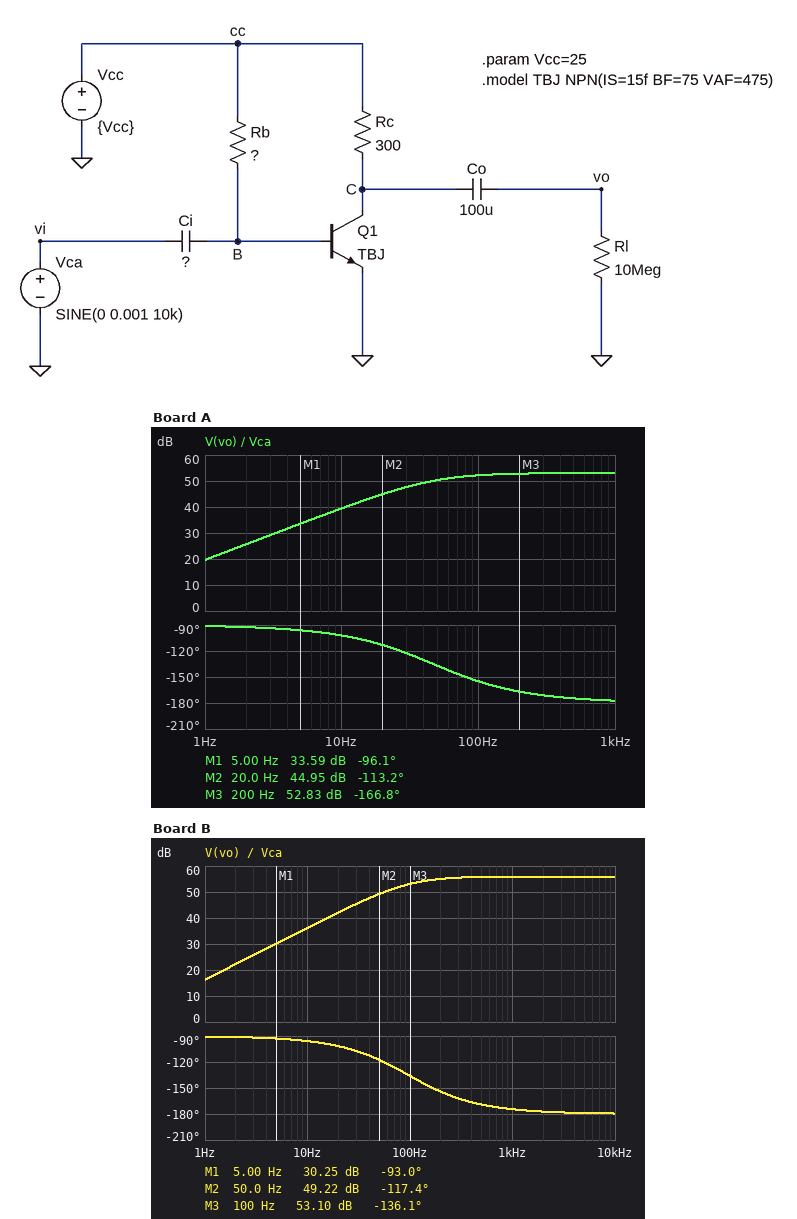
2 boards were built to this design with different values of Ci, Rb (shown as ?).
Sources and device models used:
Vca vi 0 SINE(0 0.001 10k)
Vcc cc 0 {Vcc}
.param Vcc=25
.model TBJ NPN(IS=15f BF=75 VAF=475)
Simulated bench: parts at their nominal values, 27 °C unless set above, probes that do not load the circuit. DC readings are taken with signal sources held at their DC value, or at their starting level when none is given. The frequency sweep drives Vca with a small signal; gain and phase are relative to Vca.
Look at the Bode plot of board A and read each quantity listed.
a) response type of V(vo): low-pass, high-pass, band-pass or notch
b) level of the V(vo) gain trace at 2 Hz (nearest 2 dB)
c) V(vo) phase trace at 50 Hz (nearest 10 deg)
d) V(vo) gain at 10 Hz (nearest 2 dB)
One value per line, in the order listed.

high-pass
26 dB
-140 deg
40 dB
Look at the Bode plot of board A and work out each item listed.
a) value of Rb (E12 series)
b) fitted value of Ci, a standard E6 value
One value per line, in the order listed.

47 kΩ
68 µF
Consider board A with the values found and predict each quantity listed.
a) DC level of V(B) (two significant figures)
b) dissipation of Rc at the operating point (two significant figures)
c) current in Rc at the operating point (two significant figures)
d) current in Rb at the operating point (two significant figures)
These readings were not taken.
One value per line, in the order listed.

740 mV
470 mW
40 mA
520 µA
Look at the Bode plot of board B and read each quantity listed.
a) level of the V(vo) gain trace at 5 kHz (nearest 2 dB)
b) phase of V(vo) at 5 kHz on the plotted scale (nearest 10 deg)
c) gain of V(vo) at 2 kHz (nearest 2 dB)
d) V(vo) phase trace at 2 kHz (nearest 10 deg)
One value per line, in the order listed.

56 dB
-180 deg
56 dB
-180 deg
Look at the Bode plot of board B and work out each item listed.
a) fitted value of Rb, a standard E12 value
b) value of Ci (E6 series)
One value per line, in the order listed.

33 kΩ
47 µF
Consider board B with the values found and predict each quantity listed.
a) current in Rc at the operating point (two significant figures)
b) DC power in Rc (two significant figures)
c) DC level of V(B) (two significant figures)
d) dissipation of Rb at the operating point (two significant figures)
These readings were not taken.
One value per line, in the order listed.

56 mA
940 mW
750 mV
18 mW
